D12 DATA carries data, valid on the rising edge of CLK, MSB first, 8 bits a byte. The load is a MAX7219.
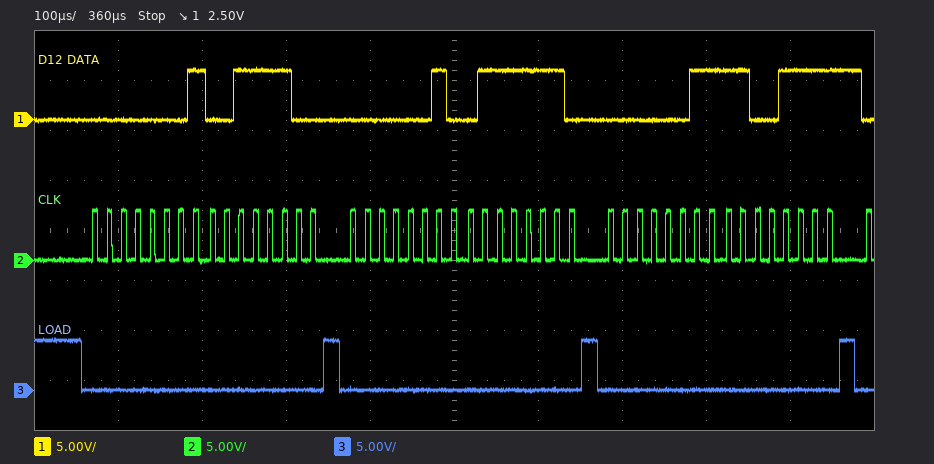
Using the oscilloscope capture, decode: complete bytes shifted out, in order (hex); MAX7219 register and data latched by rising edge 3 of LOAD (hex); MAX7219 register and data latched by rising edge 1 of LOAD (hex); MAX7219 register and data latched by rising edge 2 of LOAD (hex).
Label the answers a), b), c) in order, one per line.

a) 01 3C 02 7E 03 CF
b) register 0x3, data 0xCF
c) register 0x1, data 0x3C
d) register 0x2, data 0x7E
